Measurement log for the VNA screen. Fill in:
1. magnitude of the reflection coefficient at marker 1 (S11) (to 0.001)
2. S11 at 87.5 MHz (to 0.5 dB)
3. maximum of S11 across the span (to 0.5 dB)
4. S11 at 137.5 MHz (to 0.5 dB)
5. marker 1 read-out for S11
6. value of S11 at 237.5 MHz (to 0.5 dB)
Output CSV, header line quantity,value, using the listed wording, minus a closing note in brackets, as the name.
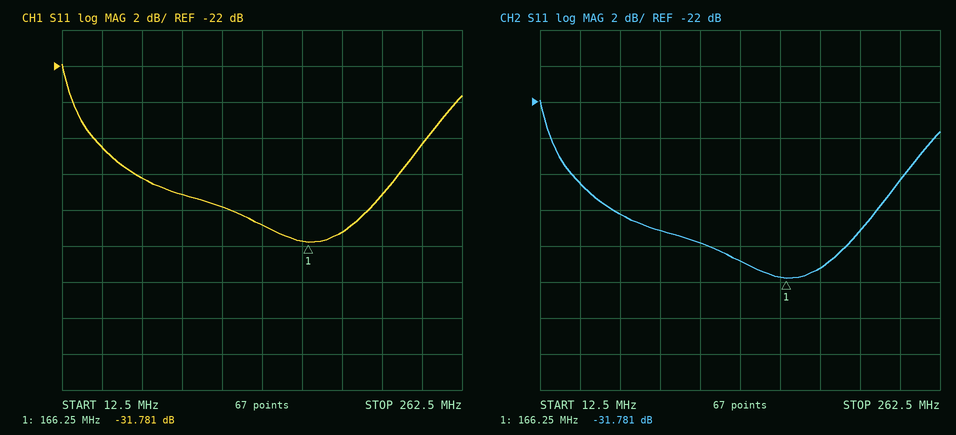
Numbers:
quantity,value
magnitude of the reflection coefficient at marker 1 (S11),0.026
S11 at 87.5 MHz,-29.0 dB
maximum of S11 across the span,-22.0 dB
S11 at 137.5 MHz,-31.0 dB
marker 1 read-out for S11,-31.781 dB
value of S11 at 237.5 MHz,-26.5 dB
